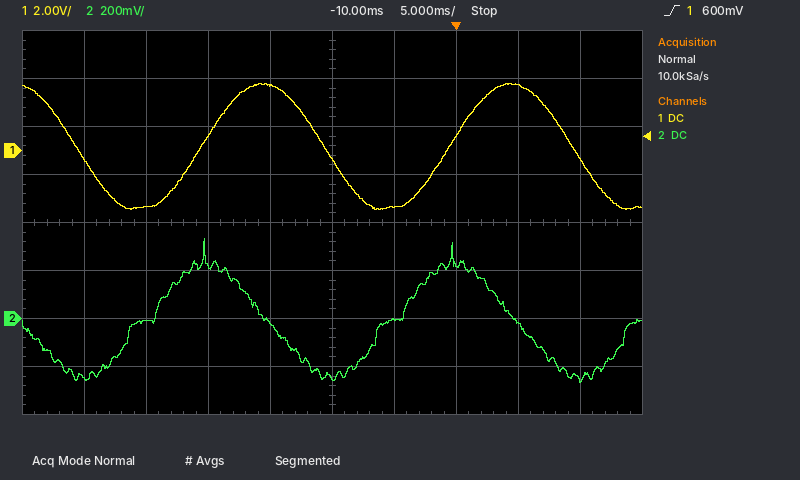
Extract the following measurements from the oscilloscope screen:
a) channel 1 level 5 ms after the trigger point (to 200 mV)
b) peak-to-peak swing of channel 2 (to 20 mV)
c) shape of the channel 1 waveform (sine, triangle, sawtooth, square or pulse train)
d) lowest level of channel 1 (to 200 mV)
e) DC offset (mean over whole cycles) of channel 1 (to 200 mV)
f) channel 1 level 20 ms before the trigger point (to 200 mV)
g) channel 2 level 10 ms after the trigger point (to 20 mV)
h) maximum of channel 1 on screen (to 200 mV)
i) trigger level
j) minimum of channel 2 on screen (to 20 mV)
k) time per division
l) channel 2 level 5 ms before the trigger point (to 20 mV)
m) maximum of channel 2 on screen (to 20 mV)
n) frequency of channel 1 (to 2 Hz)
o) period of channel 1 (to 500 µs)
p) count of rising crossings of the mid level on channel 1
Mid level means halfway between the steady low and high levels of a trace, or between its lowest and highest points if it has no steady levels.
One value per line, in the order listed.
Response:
2.8 V
600 mV
sine
-2.4 V
200 mV
600 mV
-260 mV
2.8 V
600 mV
-260 mV
5 ms
0 mV
340 mV
50 Hz
20.0 ms
2
